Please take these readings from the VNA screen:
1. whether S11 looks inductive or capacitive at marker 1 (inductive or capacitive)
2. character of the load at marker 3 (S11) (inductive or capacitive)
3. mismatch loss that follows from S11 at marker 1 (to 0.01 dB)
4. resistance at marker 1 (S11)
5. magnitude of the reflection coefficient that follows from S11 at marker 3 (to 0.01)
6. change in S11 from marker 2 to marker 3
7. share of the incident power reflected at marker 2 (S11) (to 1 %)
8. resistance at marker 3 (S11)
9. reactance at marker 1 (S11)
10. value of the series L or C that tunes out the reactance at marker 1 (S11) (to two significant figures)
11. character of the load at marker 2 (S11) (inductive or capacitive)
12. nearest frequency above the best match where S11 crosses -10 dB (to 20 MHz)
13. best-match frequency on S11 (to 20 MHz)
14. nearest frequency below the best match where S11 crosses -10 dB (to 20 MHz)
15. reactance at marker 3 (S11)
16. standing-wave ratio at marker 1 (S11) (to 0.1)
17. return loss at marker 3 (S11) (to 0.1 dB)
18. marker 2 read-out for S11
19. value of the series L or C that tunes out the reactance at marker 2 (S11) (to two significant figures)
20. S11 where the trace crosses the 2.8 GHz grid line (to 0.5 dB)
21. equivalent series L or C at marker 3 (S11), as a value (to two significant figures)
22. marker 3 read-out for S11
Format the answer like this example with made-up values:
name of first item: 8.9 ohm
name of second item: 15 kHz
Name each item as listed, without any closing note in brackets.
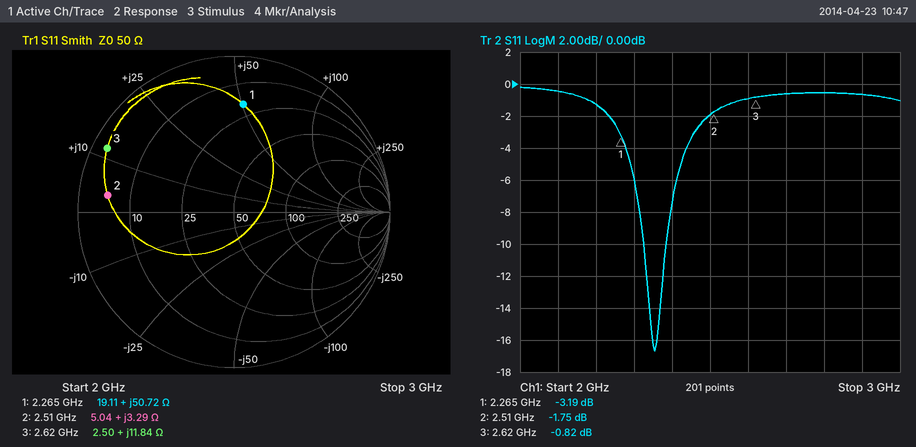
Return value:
whether S11 looks inductive or capacitive at marker 1: inductive
character of the load at marker 3 (S11): inductive
mismatch loss that follows from S11 at marker 1: 2.84 dB
resistance at marker 1: 19.11 Ω
magnitude of the reflection coefficient that follows from S11 at marker 3: 0.91
change in S11 from marker 2 to marker 3: 0.93 dB
share of the incident power reflected at marker 2 (S11): 67 %
resistance at marker 3: 2.50 Ω
reactance at marker 1: +50.72 Ω
value of the series L or C that tunes out the reactance at marker 1 (S11): 1.4 pF
character of the load at marker 2 (S11): inductive
nearest frequency above the best match where S11 crosses -10 dB: 2.38 GHz
best-match frequency on S11: 2.36 GHz
nearest frequency below the best match where S11 crosses -10 dB: 2.32 GHz
reactance at marker 3: +11.84 Ω
standing-wave ratio at marker 1 (S11): 5.5
return loss at marker 3 (S11): 0.8 dB
marker 2 read-out for S11: -1.75 dB
value of the series L or C that tunes out the reactance at marker 2 (S11): 19 pF
S11 where the trace crosses the 2.8 GHz grid line: -0.5 dB
equivalent series L or C at marker 3 (S11), as a value: 720 pH
marker 3 read-out for S11: -0.82 dB
